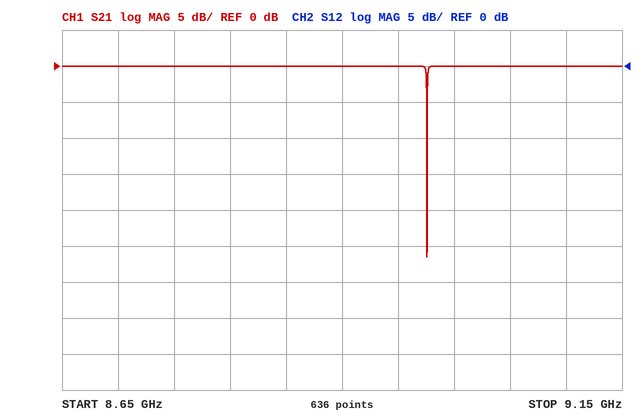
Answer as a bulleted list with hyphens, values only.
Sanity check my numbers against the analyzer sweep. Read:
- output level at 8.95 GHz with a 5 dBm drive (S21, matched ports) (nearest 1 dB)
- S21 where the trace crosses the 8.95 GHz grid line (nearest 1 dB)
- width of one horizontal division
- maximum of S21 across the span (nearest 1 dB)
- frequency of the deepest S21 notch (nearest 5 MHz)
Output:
- 5 dBm
- 0 dB
- 50 MHz
- 0 dB
- 8.975 GHz
